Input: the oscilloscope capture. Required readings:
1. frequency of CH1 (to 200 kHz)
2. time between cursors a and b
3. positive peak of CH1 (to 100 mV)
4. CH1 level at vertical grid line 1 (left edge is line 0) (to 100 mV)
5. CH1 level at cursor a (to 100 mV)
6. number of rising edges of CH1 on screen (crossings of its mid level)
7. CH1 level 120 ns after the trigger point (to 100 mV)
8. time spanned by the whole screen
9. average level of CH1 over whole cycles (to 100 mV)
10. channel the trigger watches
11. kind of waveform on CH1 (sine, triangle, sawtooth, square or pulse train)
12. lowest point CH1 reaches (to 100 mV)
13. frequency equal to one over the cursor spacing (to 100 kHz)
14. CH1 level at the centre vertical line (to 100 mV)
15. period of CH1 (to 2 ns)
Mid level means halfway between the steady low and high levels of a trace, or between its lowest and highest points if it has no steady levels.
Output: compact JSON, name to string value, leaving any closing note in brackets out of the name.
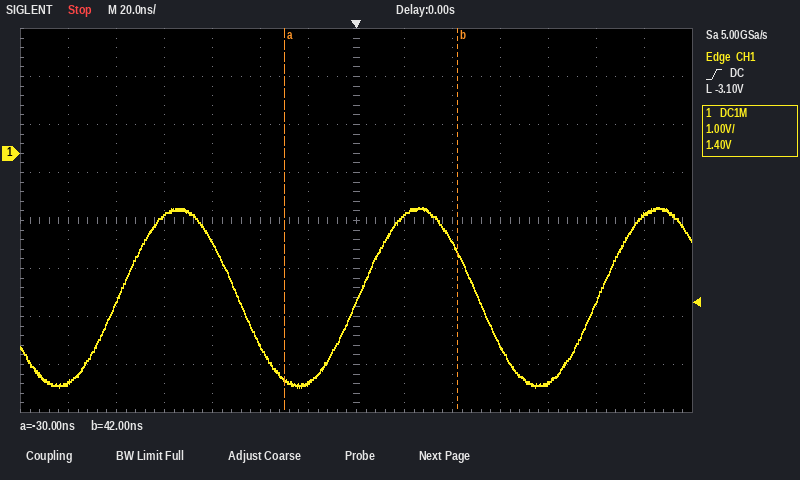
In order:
{"frequency of CH1": "10.0 MHz", "time between cursors a and b": "72 ns", "positive peak of CH1": "-1.1 V", "CH1 level at vertical grid line 1 (left edge is line 0)": "-4.8 V", "CH1 level at cursor a": "-4.7 V", "number of rising edges of CH1 on screen": "3", "CH1 level 120 ns after the trigger point": "-1.3 V", "time spanned by the whole screen": "280 ns", "average level of CH1 over whole cycles": "-3.0 V", "channel the trigger watches": "CH1", "kind of waveform on CH1": "sine", "lowest point CH1 reaches": "-4.9 V", "frequency equal to one over the cursor spacing": "13.9 MHz", "CH1 level at the centre vertical line": "-3.1 V", "period of CH1": "100 ns"}
